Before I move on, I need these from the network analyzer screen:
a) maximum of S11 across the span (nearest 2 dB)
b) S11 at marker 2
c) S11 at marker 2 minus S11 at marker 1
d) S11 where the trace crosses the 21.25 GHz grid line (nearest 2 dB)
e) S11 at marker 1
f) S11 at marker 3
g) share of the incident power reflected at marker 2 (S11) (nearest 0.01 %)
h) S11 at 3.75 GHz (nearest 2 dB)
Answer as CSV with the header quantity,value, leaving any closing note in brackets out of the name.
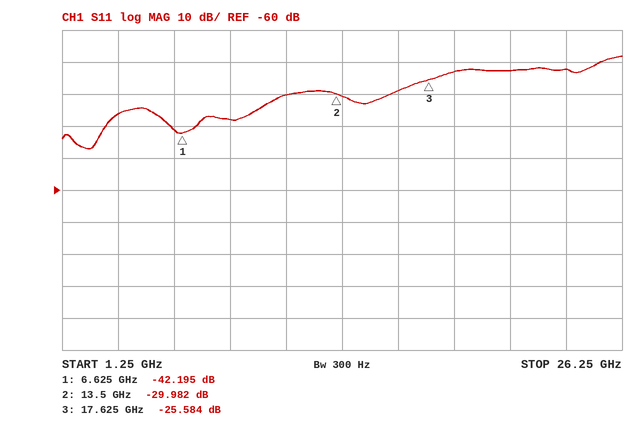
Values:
quantity,value
maximum of S11 across the span,-18 dB
S11 at marker 2,-29.982 dB
S11 at marker 2 minus S11 at marker 1,12.213 dB
S11 where the trace crosses the 21.25 GHz grid line,-22 dB
S11 at marker 1,-42.195 dB
S11 at marker 3,-25.584 dB
share of the incident power reflected at marker 2 (S11),0.10 %
S11 at 3.75 GHz,-36 dB
